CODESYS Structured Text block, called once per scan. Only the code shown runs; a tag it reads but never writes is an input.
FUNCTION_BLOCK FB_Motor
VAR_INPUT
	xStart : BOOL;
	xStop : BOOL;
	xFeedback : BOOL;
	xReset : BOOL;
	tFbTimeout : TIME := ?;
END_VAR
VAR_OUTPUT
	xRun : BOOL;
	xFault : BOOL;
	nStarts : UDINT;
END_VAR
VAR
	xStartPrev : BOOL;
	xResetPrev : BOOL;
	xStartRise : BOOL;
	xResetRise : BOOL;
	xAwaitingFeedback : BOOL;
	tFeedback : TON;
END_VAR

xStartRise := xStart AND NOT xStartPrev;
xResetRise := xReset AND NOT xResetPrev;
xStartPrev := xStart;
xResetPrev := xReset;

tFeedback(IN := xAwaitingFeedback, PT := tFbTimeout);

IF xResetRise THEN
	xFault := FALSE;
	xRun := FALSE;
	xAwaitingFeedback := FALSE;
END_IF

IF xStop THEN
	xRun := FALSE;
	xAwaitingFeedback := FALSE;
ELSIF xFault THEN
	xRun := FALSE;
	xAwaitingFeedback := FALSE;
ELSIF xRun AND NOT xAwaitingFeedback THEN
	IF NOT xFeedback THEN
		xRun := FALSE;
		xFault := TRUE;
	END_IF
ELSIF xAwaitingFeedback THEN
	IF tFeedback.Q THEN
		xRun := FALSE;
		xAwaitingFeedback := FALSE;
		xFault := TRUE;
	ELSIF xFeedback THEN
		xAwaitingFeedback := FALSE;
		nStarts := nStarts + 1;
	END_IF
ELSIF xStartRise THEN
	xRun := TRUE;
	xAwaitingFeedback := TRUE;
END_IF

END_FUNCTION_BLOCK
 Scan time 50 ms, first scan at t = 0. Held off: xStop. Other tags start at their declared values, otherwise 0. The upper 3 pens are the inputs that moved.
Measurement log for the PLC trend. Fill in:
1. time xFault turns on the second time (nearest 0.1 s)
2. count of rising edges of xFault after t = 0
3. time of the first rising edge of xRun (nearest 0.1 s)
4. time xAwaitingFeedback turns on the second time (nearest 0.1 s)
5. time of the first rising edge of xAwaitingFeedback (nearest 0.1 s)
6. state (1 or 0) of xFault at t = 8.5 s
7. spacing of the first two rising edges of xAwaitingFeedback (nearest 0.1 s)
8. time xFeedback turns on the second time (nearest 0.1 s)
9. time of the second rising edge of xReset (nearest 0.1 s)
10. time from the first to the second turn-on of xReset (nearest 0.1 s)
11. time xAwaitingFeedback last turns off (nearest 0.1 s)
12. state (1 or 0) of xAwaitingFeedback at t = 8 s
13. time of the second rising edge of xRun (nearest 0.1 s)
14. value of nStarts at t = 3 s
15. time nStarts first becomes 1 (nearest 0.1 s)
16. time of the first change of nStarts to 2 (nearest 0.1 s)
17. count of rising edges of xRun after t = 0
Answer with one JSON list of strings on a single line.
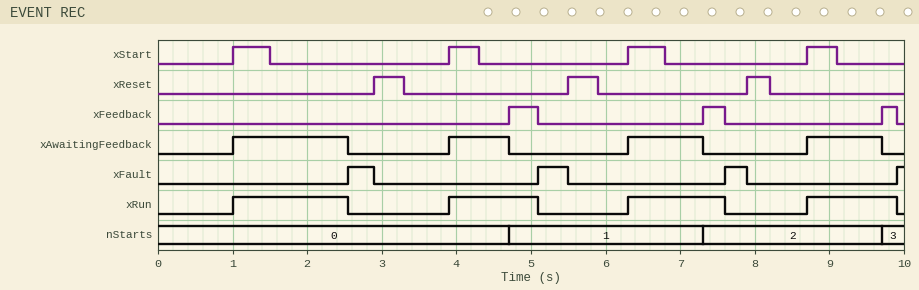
["5.1 s", "4", "1.0 s", "3.9 s", "1.0 s", "0", "2.9 s", "7.3 s", "5.5 s", "2.6 s", "9.7 s", "0", "3.9 s", "0", "4.7 s", "7.3 s", "4"]
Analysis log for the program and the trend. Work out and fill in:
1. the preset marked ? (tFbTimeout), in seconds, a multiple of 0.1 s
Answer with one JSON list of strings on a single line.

["1.5 s"]
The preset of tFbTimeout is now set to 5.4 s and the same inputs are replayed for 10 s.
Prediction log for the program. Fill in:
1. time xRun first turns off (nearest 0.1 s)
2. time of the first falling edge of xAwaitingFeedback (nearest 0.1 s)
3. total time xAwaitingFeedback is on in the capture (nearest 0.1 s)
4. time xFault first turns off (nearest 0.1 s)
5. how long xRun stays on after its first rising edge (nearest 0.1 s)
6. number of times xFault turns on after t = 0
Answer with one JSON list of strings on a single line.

["2.9 s", "2.9 s", "4.7 s", "5.5 s", "1.9 s", "3"]
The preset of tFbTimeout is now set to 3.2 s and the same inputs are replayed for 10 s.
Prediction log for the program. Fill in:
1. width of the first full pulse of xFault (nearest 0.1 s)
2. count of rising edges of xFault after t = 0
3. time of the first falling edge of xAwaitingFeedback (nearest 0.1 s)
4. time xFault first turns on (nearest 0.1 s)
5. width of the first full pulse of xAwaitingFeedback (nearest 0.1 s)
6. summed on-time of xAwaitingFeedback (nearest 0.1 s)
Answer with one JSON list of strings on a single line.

["0.4 s", "3", "2.9 s", "5.1 s", "1.9 s", "4.7 s"]
